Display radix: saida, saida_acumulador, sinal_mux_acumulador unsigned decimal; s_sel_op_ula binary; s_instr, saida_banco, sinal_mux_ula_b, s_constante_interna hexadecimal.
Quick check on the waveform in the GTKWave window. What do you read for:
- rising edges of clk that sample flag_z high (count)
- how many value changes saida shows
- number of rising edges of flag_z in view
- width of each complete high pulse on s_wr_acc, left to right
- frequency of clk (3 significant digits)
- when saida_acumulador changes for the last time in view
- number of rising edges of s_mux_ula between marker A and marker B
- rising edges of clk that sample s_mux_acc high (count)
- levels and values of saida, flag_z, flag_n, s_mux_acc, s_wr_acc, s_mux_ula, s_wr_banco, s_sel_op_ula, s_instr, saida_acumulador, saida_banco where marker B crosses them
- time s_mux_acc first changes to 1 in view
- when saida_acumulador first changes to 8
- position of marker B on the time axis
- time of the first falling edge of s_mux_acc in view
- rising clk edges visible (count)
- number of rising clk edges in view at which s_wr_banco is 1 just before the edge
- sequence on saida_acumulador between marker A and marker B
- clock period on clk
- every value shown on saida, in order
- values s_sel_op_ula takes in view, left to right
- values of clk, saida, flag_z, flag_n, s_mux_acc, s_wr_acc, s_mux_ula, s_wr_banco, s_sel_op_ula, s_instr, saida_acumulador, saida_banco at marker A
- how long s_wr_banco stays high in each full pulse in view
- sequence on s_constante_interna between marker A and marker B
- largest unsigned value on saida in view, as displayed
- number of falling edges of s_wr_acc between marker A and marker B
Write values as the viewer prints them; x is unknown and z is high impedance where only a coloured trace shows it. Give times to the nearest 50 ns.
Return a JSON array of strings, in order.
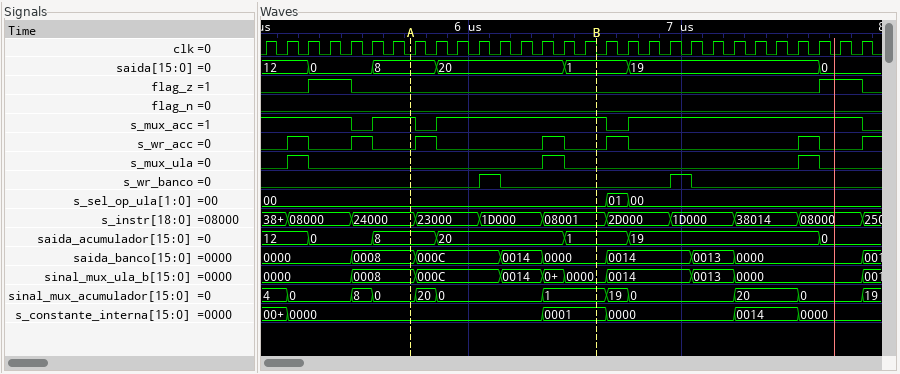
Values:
["4", "6", "2", "100 ns, 100 ns, 100 ns, 100 ns, 100 ns, 100 ns", "10.0 MHz", "7650 ns", "1", "26", "saida=1, flag_z=0, flag_n=0, s_mux_acc=1, s_wr_acc=0, s_mux_ula=0, s_wr_banco=0, s_sel_op_ula=00, s_instr=08001, saida_acumulador=1, saida_banco=0000", "5550 ns", "5550 ns", "6600 ns", "5450 ns", "29", "2", "8, 20, 1", "100 ns", "12, 0, 8, 20, 1, 19, 0", "00, 01, 00", "clk=0, saida=8, flag_z=0, flag_n=0, s_mux_acc=1, s_wr_acc=0, s_mux_ula=0, s_wr_banco=0, s_sel_op_ula=00, s_instr=24000, saida_acumulador=8, saida_banco=0008", "100 ns, 100 ns", "0000, 0001", "20", "2"]
